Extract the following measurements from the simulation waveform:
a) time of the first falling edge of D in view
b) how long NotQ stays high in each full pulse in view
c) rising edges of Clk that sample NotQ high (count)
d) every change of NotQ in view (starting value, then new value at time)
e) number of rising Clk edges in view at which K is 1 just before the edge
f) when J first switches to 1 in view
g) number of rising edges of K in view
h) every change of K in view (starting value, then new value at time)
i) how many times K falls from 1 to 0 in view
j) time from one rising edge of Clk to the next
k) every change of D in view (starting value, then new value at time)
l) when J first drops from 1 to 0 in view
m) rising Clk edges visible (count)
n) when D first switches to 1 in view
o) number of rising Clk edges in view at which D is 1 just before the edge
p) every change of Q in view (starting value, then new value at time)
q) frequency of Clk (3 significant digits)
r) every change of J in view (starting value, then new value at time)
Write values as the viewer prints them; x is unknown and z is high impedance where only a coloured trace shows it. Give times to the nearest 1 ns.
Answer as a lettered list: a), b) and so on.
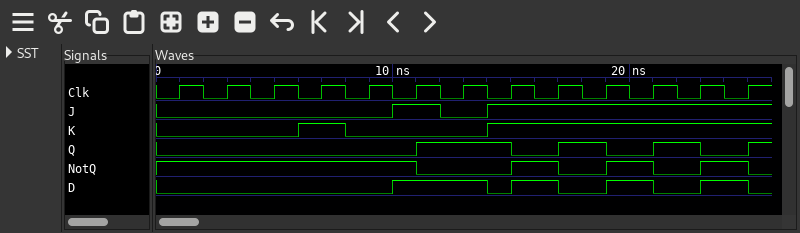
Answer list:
a) 14 ns
b) 2 ns, 2 ns, 2 ns
c) 9
d) 1, 0 at 11 ns, 1 at 15 ns, 0 at 17 ns, 1 at 19 ns, 0 at 21 ns, 1 at 23 ns, 0 at 25 ns
e) 7
f) 10 ns
g) 2
h) 0, 1 at 6 ns, 0 at 8 ns, 1 at 14 ns
i) 1
j) 2 ns
k) 0, 1 at 10 ns, 0 at 14 ns, 1 at 15 ns, 0 at 17 ns, 1 at 19 ns, 0 at 21 ns, 1 at 23 ns, 0 at 25 ns
l) 12 ns
m) 13
n) 10 ns
o) 5
p) 0, 1 at 11 ns, 0 at 15 ns, 1 at 17 ns, 0 at 19 ns, 1 at 21 ns, 0 at 23 ns, 1 at 25 ns
q) 500 MHz
r) 0, 1 at 10 ns, 0 at 12 ns, 1 at 14 ns
